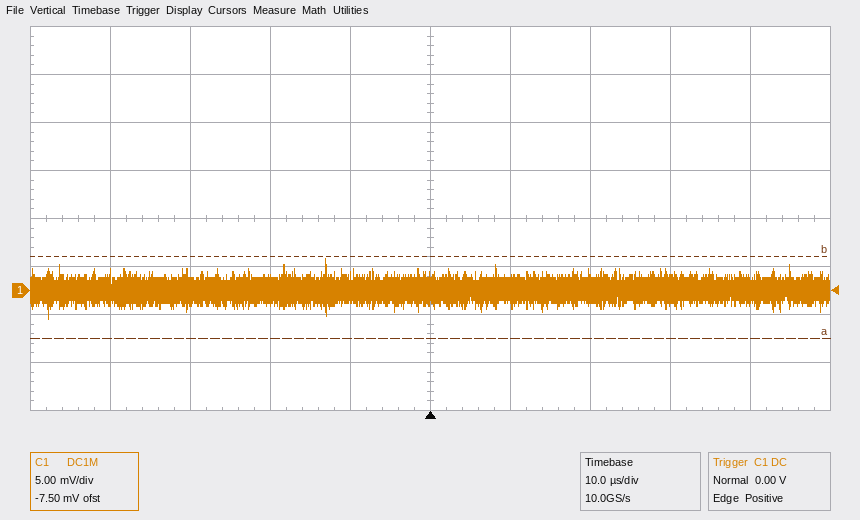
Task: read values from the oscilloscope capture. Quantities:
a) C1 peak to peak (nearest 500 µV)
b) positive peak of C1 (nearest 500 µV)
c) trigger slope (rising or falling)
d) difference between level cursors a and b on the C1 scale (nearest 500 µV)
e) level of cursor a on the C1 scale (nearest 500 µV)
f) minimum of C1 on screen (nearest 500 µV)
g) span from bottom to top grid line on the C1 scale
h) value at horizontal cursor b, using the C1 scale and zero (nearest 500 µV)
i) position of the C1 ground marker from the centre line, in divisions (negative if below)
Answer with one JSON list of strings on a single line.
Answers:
["6.5 mV", "3.5 mV", "rising", "8.5 mV", "-5.0 mV", "-3.0 mV", "40 mV", "3.5 mV", "-1.5 div"]
